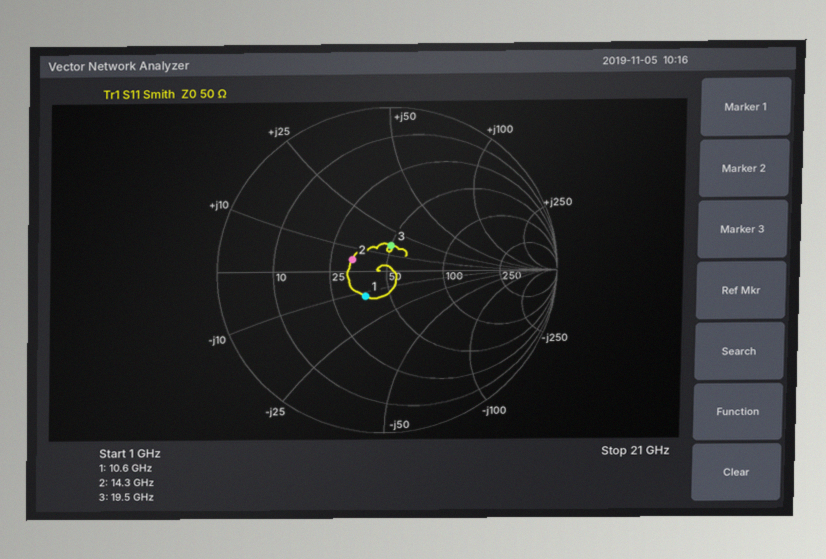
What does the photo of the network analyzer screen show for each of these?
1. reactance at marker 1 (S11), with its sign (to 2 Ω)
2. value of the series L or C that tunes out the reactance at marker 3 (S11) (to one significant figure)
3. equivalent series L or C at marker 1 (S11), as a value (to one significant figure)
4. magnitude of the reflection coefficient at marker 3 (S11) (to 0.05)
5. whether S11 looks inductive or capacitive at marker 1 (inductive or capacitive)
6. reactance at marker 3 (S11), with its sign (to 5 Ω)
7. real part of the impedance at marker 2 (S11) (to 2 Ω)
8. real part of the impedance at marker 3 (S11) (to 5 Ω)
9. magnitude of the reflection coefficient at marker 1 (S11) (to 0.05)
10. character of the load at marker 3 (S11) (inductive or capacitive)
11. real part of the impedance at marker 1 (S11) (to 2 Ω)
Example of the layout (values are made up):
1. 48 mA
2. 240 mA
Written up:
1. -12 Ω
2. 500 fF
3. 1 pF
4. 0.15
5. capacitive
6. +15 Ω
7. 32 Ω
8. 50 Ω
9. 0.20
10. inductive
11. 38 Ω
